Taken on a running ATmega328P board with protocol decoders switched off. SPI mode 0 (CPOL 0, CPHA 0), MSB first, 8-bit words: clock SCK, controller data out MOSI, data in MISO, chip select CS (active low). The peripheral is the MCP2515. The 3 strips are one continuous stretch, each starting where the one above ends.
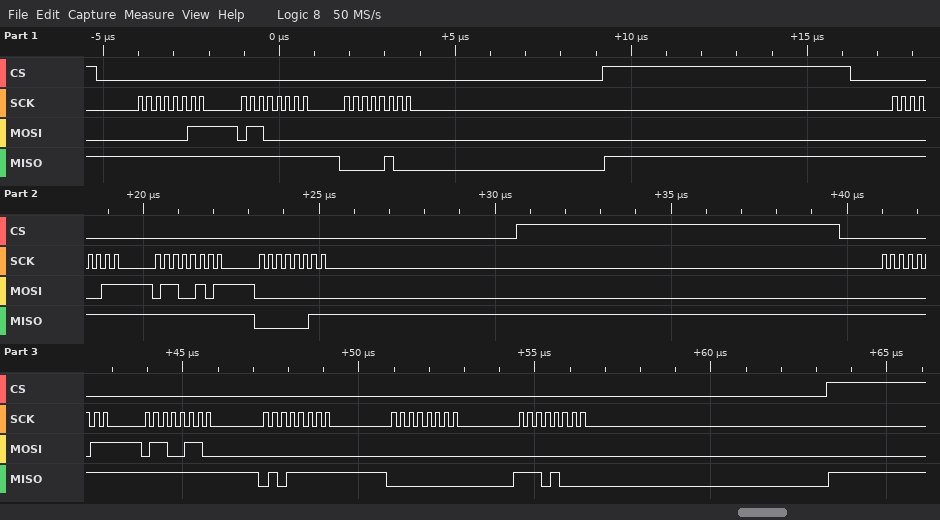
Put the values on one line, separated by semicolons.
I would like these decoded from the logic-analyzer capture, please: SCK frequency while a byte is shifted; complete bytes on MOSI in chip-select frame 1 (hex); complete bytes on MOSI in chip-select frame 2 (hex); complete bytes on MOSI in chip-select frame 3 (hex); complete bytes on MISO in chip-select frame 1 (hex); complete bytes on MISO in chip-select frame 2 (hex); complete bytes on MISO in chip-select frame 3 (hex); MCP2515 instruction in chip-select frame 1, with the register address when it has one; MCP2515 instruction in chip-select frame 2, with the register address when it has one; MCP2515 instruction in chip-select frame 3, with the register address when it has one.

4 MHz; 03 60 00; 03 65 00; 03 66 00 00 00; FF FF 04; FF FF 03; FF FF 5F 00 E8; READ 0x60; READ 0x65; READ 0x66
